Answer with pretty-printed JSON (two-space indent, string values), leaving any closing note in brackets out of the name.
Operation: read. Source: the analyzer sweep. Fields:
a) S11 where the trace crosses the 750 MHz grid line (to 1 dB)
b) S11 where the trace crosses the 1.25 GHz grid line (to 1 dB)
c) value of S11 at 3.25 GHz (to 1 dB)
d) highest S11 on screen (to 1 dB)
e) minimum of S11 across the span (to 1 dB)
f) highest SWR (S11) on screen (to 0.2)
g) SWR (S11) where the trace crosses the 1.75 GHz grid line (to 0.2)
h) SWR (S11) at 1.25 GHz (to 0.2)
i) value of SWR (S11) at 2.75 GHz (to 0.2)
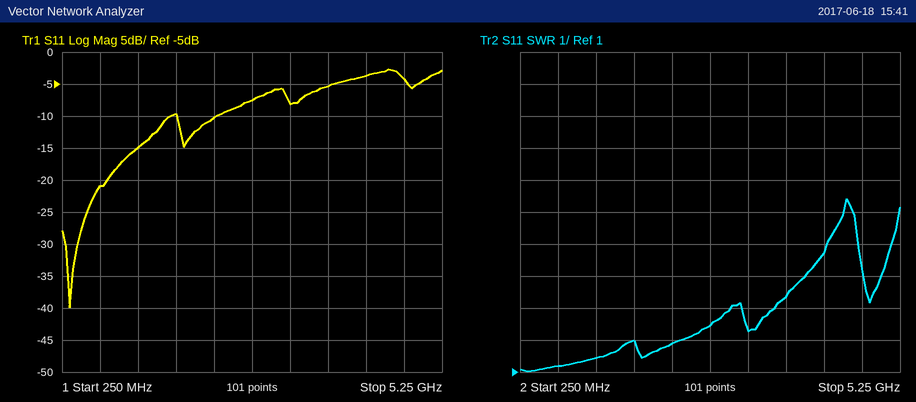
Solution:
{
  "S11 where the trace crosses the 750 MHz grid line": "-21 dB",
  "S11 where the trace crosses the 1.25 GHz grid line": "-15 dB",
  "value of S11 at 3.25 GHz": "-8 dB",
  "highest S11 on screen": "-3 dB",
  "minimum of S11 across the span": "-40 dB",
  "highest SWR (S11) on screen": "6.4",
  "SWR (S11) where the trace crosses the 1.75 GHz grid line": "2.0",
  "SWR (S11) at 1.25 GHz": "1.4",
  "value of SWR (S11) at 2.75 GHz": "2.4"
}
